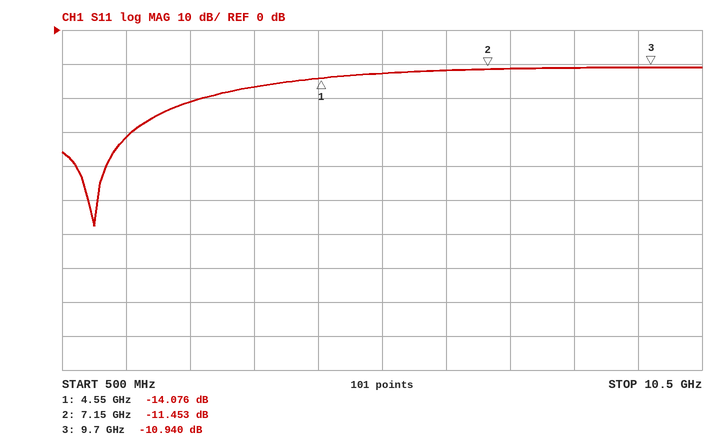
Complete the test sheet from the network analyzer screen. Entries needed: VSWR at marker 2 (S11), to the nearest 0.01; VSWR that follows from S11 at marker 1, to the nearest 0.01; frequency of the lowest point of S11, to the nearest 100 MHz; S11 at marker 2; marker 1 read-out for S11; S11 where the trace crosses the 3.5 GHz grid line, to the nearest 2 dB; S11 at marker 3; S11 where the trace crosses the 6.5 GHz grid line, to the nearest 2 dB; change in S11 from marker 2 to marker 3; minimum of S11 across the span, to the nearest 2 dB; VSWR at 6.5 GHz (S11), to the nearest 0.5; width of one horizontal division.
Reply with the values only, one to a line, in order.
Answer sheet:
1.73
1.49
1.0 GHz
-11.453 dB
-14.076 dB
-16 dB
-10.940 dB
-12 dB
0.513 dB
-58 dB
1.5
1 GHz
